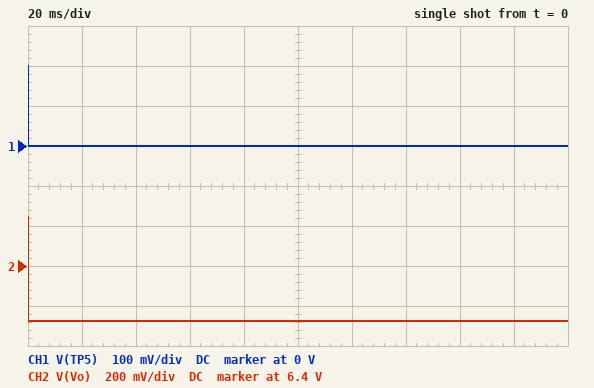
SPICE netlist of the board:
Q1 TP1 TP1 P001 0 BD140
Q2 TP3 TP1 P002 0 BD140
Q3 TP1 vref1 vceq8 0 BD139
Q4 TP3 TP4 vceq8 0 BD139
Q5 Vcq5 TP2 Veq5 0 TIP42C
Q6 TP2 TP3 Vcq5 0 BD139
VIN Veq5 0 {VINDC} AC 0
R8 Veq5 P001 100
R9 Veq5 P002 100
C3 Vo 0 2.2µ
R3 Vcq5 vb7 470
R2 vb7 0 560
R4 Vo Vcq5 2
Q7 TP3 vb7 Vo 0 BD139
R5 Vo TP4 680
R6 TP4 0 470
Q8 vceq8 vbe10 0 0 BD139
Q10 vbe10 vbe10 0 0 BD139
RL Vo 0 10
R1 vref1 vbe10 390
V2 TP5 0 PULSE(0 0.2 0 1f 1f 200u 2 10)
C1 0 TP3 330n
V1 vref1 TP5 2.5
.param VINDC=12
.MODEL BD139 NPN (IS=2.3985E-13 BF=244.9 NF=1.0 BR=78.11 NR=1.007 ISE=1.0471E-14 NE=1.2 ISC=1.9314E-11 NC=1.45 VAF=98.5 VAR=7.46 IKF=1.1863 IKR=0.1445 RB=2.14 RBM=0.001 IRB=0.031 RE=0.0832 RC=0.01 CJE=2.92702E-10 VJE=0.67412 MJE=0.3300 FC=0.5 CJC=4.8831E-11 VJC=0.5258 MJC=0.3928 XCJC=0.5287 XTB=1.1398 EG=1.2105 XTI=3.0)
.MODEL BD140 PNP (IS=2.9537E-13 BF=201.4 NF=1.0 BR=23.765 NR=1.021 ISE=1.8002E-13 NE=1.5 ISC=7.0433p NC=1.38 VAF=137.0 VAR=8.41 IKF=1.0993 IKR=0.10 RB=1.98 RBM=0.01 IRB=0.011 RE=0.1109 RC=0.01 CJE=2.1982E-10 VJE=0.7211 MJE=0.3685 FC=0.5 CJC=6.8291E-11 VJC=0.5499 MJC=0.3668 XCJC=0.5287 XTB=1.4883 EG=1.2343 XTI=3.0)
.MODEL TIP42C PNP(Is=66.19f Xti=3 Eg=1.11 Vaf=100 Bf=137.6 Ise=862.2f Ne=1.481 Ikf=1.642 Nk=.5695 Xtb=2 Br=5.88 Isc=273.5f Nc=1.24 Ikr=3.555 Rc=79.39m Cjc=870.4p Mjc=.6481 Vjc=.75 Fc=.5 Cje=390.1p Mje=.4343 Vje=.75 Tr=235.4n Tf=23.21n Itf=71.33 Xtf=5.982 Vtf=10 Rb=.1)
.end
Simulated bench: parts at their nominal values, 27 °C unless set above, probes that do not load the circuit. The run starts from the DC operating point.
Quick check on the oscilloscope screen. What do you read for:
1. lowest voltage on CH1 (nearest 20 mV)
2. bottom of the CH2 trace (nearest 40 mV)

0 V
6.12 V
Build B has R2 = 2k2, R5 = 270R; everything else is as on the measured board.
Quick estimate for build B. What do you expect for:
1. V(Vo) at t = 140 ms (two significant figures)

3.9 V
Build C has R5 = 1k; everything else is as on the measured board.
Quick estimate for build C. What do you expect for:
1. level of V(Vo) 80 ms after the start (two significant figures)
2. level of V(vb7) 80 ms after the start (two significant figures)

7.8 V
5.1 V
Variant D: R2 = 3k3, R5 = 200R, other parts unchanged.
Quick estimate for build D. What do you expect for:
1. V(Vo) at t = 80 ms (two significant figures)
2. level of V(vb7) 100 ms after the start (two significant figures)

3.6 V
3.8 V
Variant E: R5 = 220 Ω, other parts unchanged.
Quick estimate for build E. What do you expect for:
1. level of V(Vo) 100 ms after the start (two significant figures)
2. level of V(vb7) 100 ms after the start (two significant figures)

3.7 V
2.4 V
